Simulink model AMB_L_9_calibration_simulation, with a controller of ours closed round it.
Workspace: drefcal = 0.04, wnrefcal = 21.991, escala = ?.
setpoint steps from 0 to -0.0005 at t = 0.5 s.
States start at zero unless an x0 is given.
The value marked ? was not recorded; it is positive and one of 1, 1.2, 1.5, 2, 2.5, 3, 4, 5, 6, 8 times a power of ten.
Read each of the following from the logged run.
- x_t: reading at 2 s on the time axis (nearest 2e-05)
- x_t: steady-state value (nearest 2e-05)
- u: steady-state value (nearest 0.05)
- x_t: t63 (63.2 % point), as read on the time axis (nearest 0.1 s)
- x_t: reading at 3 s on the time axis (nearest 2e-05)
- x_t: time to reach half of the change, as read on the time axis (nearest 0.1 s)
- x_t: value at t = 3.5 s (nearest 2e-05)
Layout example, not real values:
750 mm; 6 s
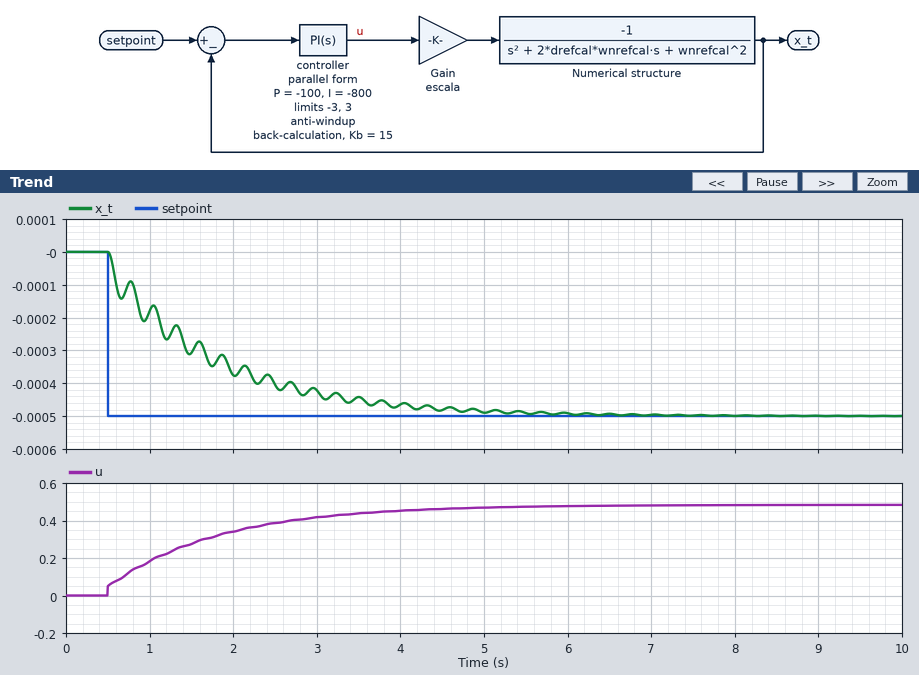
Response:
-0.00038; -0.00050; 0.50; 1.7 s; -0.00042; 1.2 s; -0.00044
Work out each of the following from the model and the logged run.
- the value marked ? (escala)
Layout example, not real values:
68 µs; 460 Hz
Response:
0.5
